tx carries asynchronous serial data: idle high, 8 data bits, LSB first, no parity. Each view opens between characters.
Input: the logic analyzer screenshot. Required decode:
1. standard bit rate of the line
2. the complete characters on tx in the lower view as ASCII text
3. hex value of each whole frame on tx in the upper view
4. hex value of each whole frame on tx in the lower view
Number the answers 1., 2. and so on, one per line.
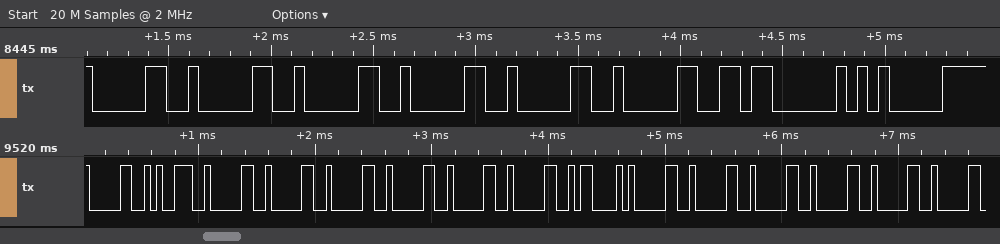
1. 19200 baud
2. "09000000C00000"
3. 30, 30, 30, 30, 30, 30, 03, 05
4. 30, 39, 30, 30, 30, 30, 30, 30, 43, 30, 30, 30, 30, 30
